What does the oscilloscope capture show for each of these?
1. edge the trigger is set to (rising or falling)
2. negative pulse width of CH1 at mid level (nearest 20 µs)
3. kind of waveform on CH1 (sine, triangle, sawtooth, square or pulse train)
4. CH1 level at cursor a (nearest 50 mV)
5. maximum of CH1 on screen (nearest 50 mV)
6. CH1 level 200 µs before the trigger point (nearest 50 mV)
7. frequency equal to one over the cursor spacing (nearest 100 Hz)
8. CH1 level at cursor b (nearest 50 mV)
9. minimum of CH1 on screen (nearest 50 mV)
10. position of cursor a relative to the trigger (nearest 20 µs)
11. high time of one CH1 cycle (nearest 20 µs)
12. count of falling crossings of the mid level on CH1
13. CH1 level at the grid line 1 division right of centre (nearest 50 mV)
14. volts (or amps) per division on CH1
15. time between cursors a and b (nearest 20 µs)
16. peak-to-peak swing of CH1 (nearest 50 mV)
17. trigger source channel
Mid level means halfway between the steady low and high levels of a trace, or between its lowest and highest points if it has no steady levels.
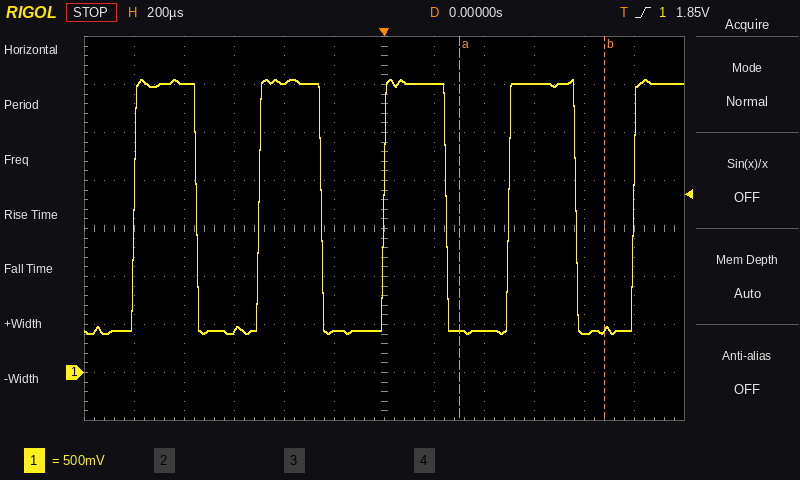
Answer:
rising
240 µs
square
450 mV
3.05 V
450 mV
1.7 kHz
450 mV
400 mV
+300 µs
260 µs
4
3.00 V
500 mV
580 µs
2.65 V
CH1
